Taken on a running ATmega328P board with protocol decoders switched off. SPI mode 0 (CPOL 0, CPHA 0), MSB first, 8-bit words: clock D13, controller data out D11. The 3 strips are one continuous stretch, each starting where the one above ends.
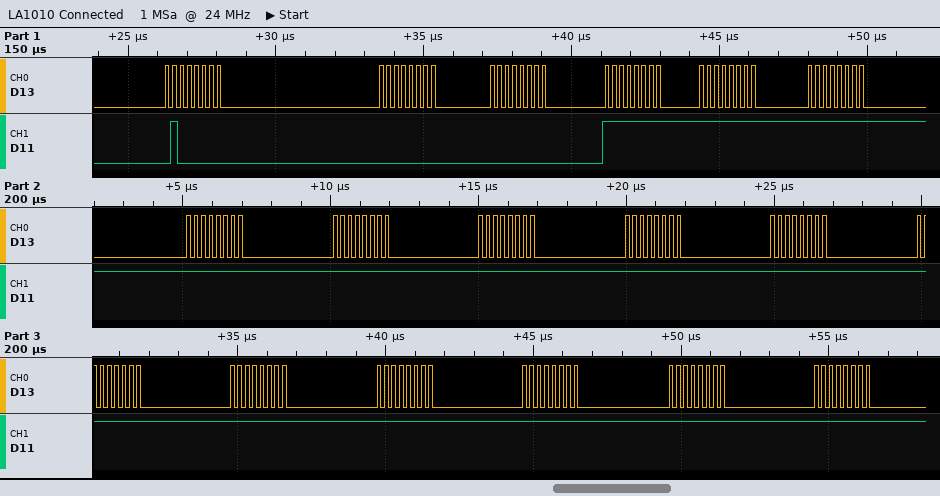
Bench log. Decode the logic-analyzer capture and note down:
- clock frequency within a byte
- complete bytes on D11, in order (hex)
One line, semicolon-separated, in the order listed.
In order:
4 MHz; 0x40 0x00 0x00 0xFF 0xFF 0xFF 0xFF 0xFF 0xFF 0xFF 0xFF 0xFF 0xFF 0xFF 0xFF 0xFF 0xFF
